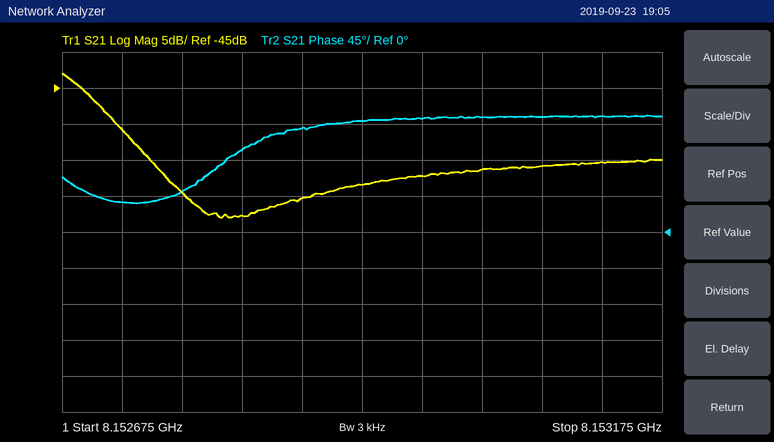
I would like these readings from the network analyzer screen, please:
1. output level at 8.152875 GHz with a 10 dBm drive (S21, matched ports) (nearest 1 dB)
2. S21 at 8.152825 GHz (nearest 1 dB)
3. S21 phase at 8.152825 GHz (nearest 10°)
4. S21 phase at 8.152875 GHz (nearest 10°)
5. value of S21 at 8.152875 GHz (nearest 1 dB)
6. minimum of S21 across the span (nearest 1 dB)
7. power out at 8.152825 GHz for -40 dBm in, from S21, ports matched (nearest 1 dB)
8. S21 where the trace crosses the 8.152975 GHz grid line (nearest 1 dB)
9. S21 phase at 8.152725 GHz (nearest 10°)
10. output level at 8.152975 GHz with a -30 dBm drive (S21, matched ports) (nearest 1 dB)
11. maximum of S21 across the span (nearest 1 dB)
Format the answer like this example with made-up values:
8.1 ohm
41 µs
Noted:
-50 dBm
-63 dB
100°
130°
-60 dB
-63 dB
-103 dBm
-57 dB
40°
-87 dBm
-43 dB
